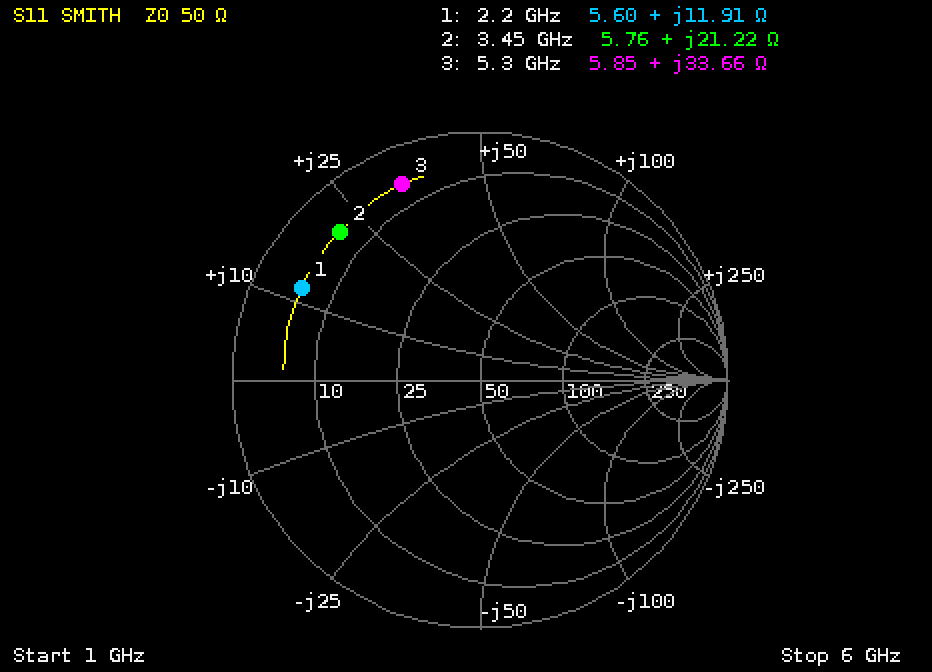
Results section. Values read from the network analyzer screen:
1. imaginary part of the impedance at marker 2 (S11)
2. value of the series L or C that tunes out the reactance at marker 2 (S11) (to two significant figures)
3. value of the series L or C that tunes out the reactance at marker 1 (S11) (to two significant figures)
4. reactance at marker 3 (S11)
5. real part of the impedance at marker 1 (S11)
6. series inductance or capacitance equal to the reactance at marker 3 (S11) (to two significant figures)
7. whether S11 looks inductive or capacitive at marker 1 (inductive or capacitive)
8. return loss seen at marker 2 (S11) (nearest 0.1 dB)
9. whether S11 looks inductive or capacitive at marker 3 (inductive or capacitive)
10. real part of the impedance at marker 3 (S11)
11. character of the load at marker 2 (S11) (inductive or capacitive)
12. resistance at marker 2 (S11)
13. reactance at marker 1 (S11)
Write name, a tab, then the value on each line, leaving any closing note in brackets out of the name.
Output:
imaginary part of the impedance at marker 2	+21.22 Ω
value of the series L or C that tunes out the reactance at marker 2 (S11)	2.2 pF
value of the series L or C that tunes out the reactance at marker 1 (S11)	6.1 pF
reactance at marker 3	+33.66 Ω
real part of the impedance at marker 1	5.60 Ω
series inductance or capacitance equal to the reactance at marker 3 (S11)	1.0 nH
whether S11 looks inductive or capacitive at marker 1	inductive
return loss seen at marker 2 (S11)	1.7 dB
whether S11 looks inductive or capacitive at marker 3	inductive
real part of the impedance at marker 3	5.85 Ω
character of the load at marker 2 (S11)	inductive
resistance at marker 2	5.76 Ω
reactance at marker 1	+11.91 Ω
